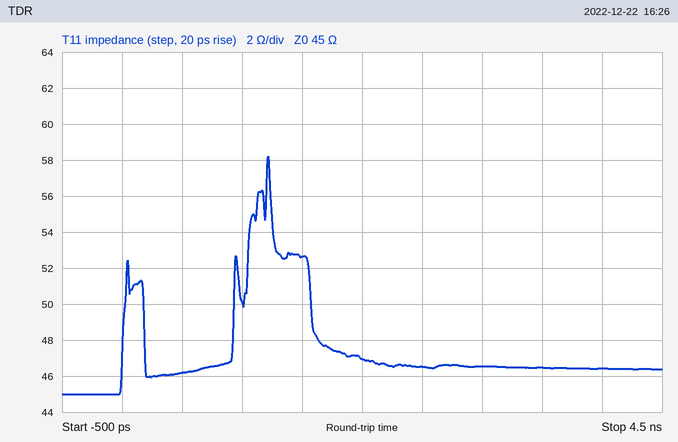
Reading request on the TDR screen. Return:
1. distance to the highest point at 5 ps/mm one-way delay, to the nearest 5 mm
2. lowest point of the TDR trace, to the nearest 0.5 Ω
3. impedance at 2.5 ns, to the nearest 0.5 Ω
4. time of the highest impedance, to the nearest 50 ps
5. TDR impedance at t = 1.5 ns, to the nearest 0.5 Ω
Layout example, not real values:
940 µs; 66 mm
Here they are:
120 mm; 45.0 Ω; 46.5 Ω; 1.20 ns; 52.5 Ω
